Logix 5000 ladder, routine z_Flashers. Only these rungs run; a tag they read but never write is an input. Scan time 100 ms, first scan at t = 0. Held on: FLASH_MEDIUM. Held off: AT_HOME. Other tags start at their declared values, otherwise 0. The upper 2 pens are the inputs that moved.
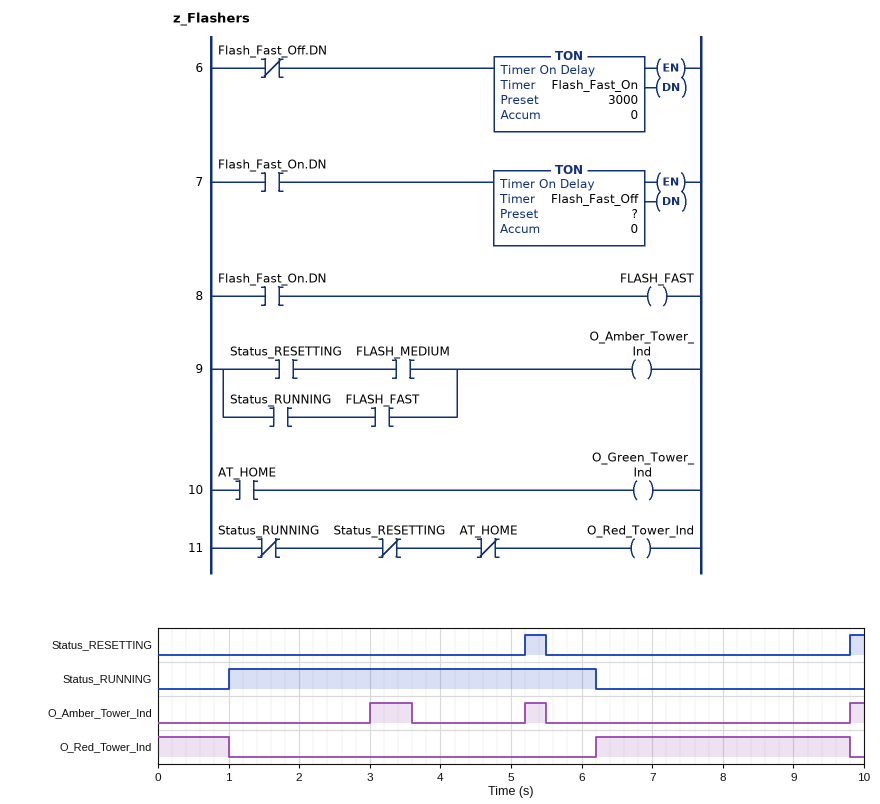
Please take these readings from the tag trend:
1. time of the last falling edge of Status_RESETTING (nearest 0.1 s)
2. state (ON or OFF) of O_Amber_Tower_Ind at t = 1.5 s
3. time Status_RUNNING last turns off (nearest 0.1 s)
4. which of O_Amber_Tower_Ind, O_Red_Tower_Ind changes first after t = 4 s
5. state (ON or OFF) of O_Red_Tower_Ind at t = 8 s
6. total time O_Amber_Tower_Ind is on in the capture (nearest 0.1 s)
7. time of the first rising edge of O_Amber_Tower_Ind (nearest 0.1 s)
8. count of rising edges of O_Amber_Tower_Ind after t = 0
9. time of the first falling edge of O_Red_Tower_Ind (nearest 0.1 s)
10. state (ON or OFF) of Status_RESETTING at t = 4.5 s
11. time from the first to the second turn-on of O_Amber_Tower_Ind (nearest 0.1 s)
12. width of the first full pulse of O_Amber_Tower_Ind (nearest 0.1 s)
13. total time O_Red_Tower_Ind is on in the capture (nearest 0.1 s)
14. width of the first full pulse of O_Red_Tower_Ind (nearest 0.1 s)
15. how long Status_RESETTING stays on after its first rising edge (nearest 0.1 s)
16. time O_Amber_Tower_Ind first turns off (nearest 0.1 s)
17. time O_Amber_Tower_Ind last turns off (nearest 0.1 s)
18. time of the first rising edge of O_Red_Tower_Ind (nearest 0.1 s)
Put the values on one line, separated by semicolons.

5.5 s; OFF; 6.2 s; O_Amber_Tower_Ind; ON; 1.1 s; 3.0 s; 3; 1.0 s; OFF; 2.2 s; 0.6 s; 4.6 s; 3.6 s; 0.3 s; 3.6 s; 5.5 s; 6.2 s
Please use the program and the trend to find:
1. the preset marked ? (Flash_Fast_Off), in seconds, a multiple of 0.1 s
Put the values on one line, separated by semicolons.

0.5 s
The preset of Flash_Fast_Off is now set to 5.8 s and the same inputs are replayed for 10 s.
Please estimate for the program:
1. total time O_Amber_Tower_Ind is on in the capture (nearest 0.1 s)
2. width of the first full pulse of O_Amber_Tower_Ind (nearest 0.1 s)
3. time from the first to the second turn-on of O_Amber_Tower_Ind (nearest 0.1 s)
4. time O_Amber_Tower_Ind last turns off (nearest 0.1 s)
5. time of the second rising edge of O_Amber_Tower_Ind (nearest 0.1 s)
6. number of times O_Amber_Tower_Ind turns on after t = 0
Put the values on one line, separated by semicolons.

3.4 s; 3.2 s; 6.8 s; 6.2 s; 9.8 s; 2
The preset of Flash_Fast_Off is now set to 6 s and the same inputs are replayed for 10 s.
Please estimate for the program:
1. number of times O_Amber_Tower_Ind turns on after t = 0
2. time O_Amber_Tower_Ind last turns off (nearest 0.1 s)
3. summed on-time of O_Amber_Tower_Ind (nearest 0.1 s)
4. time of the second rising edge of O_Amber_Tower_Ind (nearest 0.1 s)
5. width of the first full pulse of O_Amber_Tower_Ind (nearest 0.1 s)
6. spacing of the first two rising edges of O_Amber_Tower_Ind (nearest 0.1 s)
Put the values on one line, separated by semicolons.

2; 6.2 s; 3.4 s; 9.8 s; 3.2 s; 6.8 s
